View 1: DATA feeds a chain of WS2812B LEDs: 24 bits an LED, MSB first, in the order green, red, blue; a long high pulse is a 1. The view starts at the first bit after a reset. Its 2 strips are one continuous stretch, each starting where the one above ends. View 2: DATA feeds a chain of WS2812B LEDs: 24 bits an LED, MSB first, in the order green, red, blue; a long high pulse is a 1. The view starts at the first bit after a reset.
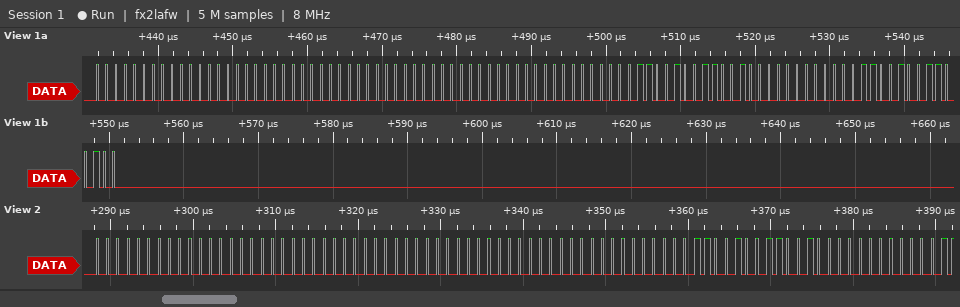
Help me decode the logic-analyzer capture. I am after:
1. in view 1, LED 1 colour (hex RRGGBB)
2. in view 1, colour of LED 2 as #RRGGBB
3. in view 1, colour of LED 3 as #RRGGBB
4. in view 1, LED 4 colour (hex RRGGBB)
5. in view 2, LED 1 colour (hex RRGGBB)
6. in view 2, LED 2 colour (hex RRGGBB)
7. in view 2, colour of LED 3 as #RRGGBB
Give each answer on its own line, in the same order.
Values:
#000000
#000000
#320064
#320064
#000000
#000000
#320064
